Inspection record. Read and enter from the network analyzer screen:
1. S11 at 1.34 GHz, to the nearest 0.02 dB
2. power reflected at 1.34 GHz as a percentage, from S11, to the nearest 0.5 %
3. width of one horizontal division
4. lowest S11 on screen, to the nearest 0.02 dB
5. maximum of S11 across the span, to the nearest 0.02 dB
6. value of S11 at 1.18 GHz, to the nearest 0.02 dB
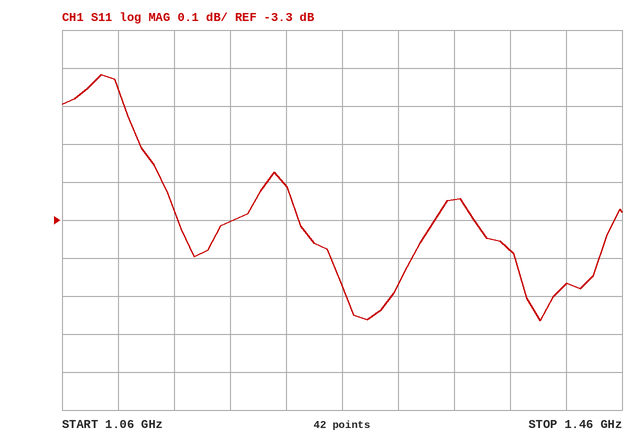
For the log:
-3.24 dB
47.5 %
40 MHz
-3.56 dB
-2.92 dB
-3.30 dB
